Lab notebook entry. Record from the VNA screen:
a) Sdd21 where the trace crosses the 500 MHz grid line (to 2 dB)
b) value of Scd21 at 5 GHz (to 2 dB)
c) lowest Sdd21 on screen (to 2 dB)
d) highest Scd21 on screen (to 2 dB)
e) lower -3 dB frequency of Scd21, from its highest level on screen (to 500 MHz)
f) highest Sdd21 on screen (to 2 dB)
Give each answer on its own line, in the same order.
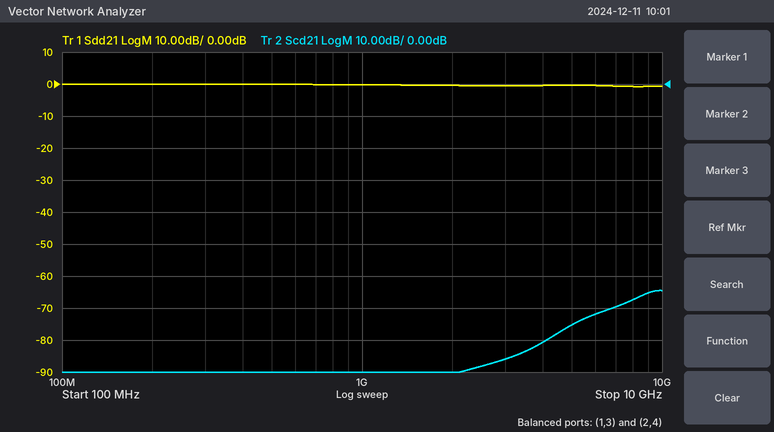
0 dB
-76 dB
0 dB
-64 dB
8.0 GHz
0 dB
